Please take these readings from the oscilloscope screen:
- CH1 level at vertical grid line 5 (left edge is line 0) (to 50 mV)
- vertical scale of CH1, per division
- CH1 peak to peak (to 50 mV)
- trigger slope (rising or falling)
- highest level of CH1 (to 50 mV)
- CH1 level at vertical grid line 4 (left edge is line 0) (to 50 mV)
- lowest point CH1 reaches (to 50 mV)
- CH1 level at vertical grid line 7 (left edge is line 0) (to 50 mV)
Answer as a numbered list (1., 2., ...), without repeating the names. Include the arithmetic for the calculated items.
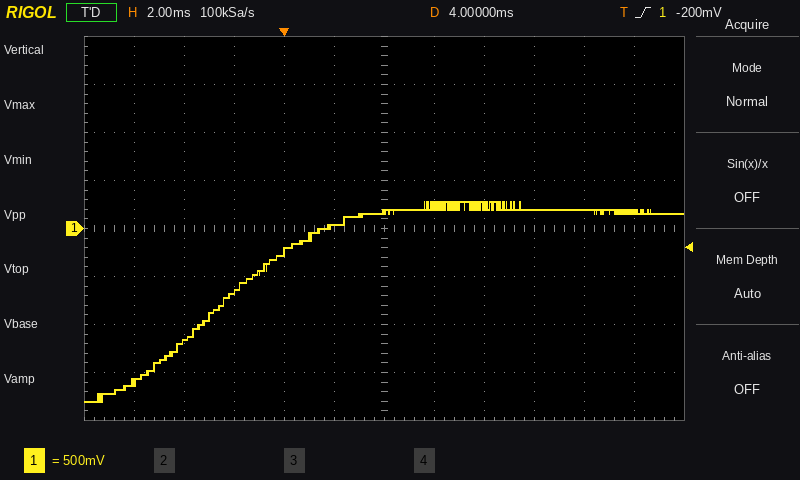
1. 50 mV
2. 500 mV
3. 300 mV − (-1.80 V) = 2.10 V
4. rising
5. 300 mV
6. -250 mV
7. -1.80 V
8. 250 mV
